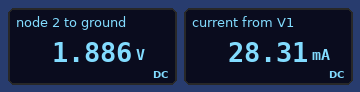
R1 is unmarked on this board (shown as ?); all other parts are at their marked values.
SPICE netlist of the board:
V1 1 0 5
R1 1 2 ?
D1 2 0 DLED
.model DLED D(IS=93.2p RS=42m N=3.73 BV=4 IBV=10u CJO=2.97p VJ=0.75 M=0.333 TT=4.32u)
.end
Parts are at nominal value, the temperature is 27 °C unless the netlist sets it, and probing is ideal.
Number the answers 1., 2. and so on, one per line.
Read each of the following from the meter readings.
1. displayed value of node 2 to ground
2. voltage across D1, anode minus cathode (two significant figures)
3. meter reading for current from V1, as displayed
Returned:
1. 1.886 V
2. 1.9 V
3. 28.31 mA
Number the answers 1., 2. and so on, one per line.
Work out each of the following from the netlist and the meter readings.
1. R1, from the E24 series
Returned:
1. 110 Ω
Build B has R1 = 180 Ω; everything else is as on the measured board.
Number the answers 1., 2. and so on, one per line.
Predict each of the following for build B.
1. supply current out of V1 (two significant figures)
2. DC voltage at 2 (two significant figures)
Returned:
1. 18 mA
2. 1.8 V
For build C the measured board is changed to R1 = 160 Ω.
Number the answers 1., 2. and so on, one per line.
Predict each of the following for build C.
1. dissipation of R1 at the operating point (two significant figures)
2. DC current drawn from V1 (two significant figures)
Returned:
1. 62 mW
2. 20 mA
